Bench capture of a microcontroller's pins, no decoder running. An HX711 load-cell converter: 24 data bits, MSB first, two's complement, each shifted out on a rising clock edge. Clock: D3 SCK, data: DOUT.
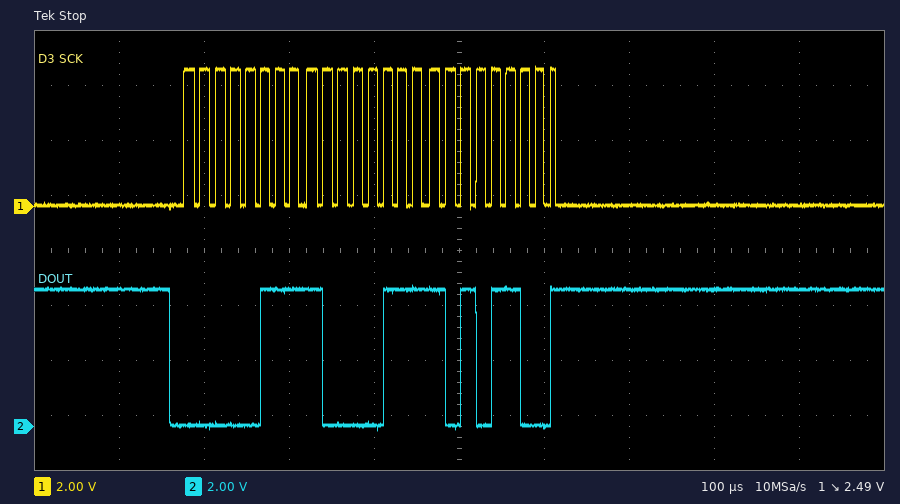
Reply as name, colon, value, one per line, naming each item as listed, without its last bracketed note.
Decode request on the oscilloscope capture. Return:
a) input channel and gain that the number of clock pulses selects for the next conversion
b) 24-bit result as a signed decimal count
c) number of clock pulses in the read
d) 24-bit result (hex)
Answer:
input channel and gain that the number of clock pulses selects for the next conversion: channel A, gain 128
24-bit result as a signed decimal count: 493484
number of clock pulses in the read: 25
24-bit result: 0x0787AC
